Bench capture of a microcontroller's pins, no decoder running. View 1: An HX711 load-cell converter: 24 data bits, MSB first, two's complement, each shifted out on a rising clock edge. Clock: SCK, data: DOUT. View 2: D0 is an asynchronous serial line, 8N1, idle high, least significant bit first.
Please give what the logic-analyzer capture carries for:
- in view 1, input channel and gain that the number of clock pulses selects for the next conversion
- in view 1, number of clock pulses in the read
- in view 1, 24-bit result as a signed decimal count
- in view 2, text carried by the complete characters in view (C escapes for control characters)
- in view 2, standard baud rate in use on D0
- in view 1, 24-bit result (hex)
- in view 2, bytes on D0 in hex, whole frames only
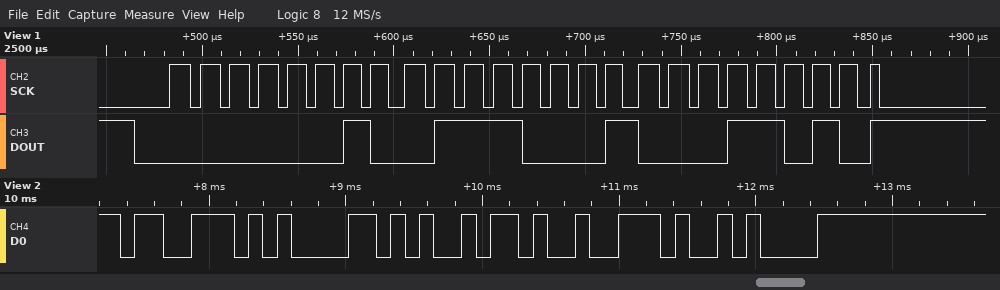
channel A, gain 128
25
160026
"sair\n"
9600 baud
0x02711A
0x73 0x61 0x69 0x72 0x0A
